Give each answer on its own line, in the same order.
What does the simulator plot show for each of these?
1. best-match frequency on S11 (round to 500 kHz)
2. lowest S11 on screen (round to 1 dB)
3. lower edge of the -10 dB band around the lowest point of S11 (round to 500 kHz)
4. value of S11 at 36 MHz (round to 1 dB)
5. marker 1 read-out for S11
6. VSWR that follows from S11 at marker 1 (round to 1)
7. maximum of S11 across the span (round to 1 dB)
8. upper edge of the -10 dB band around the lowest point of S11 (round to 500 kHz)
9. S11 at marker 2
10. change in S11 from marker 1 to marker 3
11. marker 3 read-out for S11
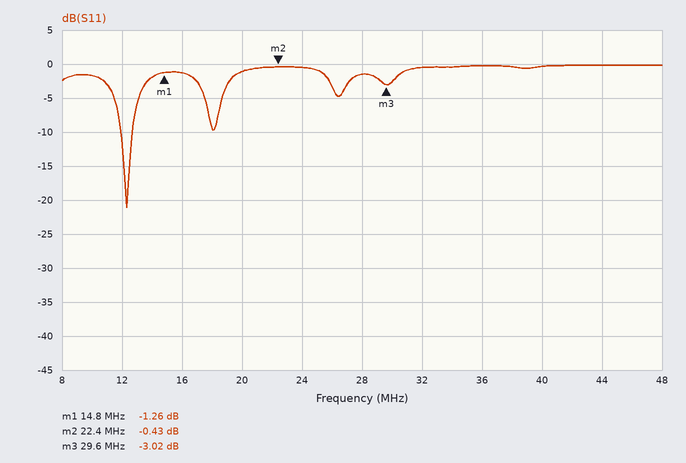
12.5 MHz
-21 dB
12.0 MHz
0 dB
-1.26 dB
14
0 dB
12.5 MHz
-0.43 dB
-1.76 dB
-3.02 dB
